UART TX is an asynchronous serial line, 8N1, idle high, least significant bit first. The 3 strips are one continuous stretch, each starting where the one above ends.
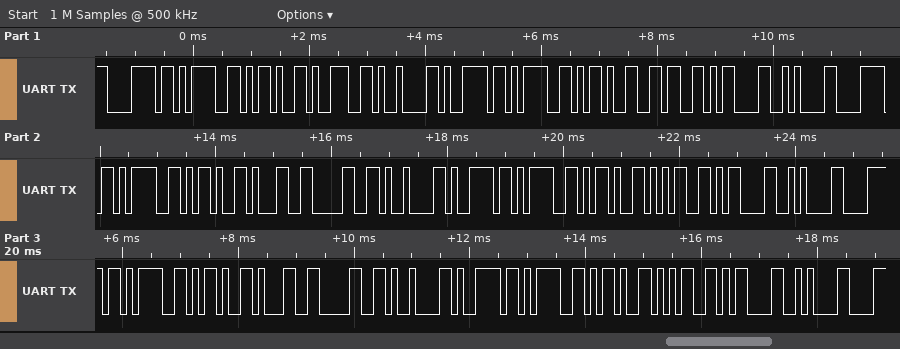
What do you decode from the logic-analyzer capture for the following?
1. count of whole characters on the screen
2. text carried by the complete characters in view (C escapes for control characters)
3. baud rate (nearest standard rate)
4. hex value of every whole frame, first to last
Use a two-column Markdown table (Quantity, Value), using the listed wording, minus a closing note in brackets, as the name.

| Quantity | Value |
|---|---|
| count of whole characters on the screen | 35 |
| text carried by the complete characters in view | "x=-9\ty=-6\r\nx=-10\ty=-5\r\nx=-10\ty=-5\r\n" |
| baud rate | 9600 baud |
| hex value of every whole frame, first to last | 78 3D 2D 39 09 79 3D 2D 36 0D 0A 78 3D 2D 31 30 09 79 3D 2D 35 0D 0A 78 3D 2D 31 30 09 79 3D 2D 35 0D 0A |
